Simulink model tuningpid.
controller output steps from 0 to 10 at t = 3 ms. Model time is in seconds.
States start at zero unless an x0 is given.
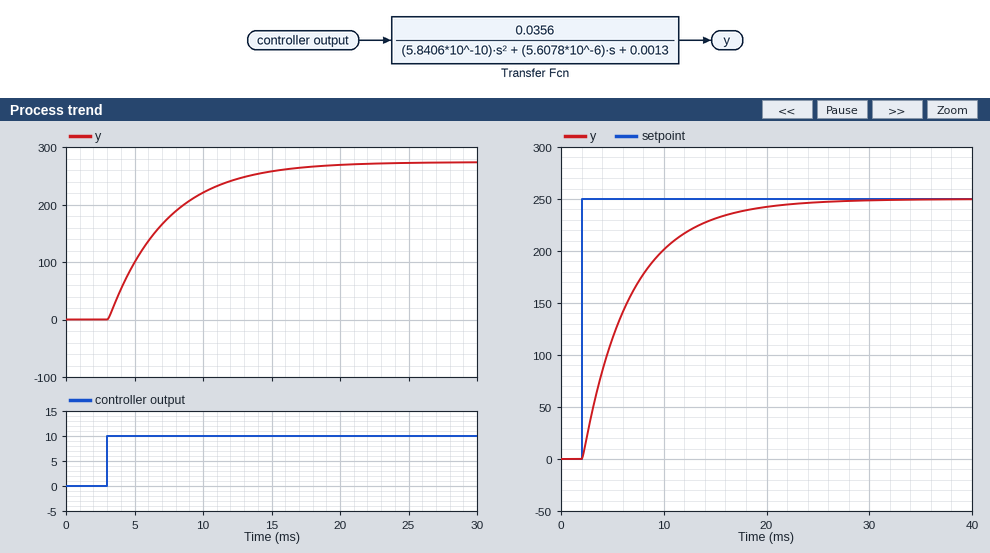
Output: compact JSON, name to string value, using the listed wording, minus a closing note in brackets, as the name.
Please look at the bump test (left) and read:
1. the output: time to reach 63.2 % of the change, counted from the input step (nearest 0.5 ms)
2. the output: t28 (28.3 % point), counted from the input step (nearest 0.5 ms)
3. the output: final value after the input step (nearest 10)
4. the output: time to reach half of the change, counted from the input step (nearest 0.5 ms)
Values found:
{"the output: time to reach 63.2 % of the change, counted from the input step": "4.5 ms", "the output: t28 (28.3 % point), counted from the input step": "1.5 ms", "the output: final value after the input step": "270", "the output: time to reach half of the change, counted from the input step": "3.0 ms"}
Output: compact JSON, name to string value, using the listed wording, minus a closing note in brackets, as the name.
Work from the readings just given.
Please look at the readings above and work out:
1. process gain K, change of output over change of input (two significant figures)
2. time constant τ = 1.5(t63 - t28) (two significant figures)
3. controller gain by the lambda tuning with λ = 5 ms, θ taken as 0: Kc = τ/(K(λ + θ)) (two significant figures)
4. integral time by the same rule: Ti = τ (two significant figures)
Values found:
{"process gain K, change of output over change of input": "27", "time constant τ = 1.5(t63 - t28)": "4.5 ms", "controller gain by the lambda tuning with λ = 5 ms, θ taken as 0: Kc = τ/(K(λ + θ))": "0.033", "integral time by the same rule: Ti = τ": "4.5 ms"}
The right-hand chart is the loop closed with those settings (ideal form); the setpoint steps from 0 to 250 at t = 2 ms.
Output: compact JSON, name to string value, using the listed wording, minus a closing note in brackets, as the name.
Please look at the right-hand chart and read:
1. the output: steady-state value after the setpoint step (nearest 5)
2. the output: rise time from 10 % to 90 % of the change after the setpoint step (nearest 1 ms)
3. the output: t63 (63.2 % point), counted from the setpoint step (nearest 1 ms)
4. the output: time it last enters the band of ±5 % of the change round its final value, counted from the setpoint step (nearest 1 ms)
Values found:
{"the output: steady-state value after the setpoint step": "250", "the output: rise time from 10 % to 90 % of the change after the setpoint step": "11 ms", "the output: t63 (63.2 % point), counted from the setpoint step": "5 ms", "the output: time it last enters the band of ±5 % of the change round its final value, counted from the setpoint step": "15 ms"}
